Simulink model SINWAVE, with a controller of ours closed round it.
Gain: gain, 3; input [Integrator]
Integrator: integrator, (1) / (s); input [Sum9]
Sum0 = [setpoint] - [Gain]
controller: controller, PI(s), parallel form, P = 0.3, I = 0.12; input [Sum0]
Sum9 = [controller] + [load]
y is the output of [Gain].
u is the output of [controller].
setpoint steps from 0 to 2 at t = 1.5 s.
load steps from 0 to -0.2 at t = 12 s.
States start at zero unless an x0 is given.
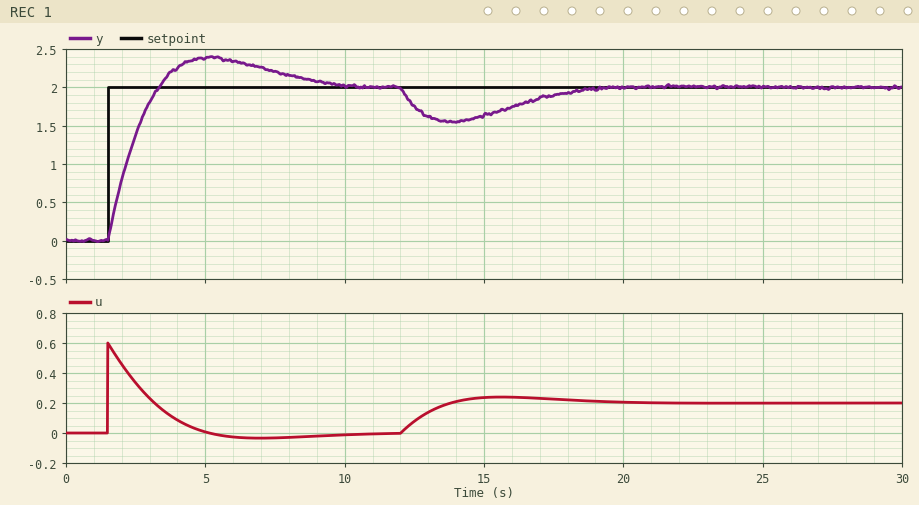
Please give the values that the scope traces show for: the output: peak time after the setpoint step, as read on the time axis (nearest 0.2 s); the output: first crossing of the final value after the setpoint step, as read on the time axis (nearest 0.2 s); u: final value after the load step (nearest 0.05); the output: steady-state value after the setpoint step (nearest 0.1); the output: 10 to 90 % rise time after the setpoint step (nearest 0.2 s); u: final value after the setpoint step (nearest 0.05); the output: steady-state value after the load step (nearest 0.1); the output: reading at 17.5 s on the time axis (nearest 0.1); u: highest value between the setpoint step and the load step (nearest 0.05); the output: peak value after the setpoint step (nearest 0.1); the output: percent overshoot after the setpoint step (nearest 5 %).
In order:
5.2 s
3.4 s
0.20
2.0
1.4 s
0.00
2.0
1.9
0.60
2.4
20 %
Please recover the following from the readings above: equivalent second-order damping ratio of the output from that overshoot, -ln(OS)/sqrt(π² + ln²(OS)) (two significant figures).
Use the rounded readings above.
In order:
0.46
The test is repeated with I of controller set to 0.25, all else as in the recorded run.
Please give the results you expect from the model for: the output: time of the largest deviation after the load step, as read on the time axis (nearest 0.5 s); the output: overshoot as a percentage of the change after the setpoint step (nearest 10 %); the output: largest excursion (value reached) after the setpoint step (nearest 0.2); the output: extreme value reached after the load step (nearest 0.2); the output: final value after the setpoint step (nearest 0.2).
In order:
13.5 s
30 %
2.6
1.6
2.0
